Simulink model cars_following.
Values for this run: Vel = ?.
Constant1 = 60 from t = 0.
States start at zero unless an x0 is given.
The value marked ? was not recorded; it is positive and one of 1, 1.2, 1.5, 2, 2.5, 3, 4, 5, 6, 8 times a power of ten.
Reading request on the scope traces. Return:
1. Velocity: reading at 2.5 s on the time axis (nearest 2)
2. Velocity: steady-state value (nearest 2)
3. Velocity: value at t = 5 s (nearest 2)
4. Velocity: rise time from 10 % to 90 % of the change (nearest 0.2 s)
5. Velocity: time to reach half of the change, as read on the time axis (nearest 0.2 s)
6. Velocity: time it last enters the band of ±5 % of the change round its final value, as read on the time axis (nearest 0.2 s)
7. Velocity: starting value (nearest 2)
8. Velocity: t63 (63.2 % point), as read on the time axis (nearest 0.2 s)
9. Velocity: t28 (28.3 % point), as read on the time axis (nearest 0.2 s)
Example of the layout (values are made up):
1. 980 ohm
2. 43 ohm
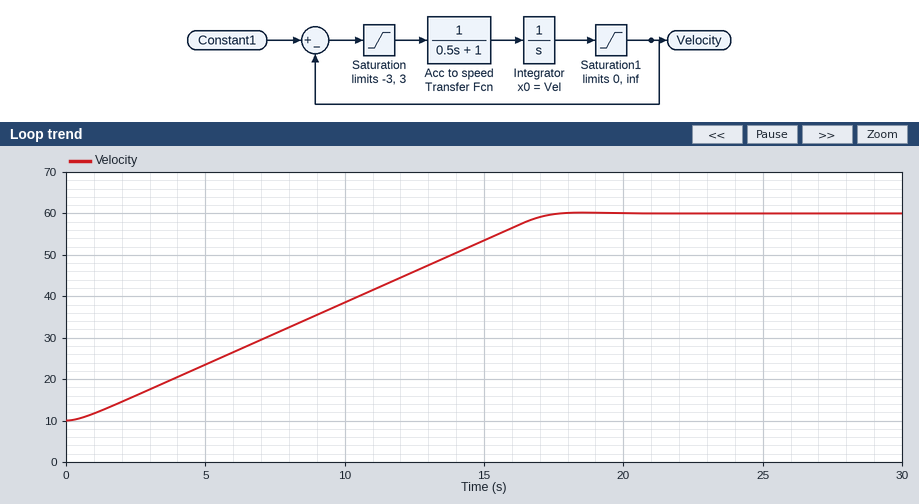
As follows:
1. 16
2. 60
3. 24
4. 13.4 s
5. 8.8 s
6. 16.4 s
7. 10
8. 11.0 s
9. 5.2 s
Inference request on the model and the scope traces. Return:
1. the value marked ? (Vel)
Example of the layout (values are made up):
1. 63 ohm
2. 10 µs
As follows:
1. 10
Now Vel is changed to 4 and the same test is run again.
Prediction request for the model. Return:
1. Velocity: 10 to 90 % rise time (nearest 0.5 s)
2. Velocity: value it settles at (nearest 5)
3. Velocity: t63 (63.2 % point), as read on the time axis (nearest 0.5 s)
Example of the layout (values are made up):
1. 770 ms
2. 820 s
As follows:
1. 15.0 s
2. 60
3. 12.5 s
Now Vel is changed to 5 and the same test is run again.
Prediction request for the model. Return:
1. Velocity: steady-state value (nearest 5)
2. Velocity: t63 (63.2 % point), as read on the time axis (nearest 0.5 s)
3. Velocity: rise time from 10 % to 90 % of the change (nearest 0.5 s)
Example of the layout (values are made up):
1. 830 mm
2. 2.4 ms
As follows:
1. 60
2. 12.0 s
3. 14.5 s
